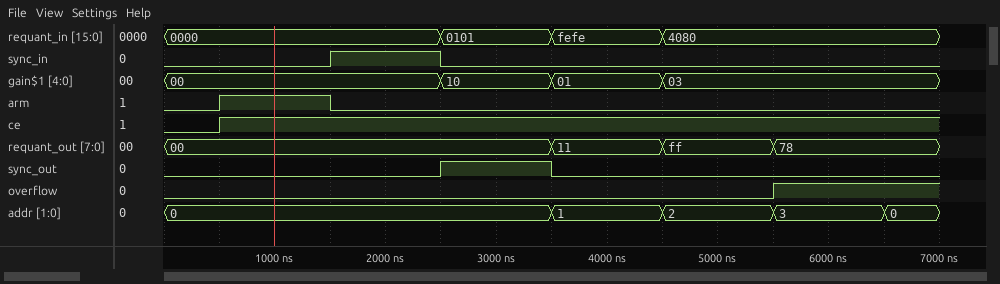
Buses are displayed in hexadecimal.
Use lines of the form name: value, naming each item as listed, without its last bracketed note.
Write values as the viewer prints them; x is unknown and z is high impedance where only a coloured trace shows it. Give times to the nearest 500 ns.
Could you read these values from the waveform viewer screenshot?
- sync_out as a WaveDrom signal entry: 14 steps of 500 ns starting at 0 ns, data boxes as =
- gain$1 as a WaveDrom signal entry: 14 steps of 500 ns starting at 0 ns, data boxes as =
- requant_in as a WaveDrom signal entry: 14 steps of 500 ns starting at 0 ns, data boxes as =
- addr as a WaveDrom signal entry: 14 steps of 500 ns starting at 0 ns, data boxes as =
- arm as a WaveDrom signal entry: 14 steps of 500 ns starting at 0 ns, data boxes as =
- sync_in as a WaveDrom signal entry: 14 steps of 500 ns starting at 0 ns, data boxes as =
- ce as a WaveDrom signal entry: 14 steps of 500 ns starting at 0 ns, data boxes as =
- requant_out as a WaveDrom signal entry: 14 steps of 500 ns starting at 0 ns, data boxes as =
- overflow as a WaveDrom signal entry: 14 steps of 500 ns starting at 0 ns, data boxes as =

sync_out as a WaveDrom signal entry: 14 steps of 500 ns starting at 0 ns, data boxes as =: {name: 'sync_out', wave: '0....1.0......'}
gain$1 as a WaveDrom signal entry: 14 steps of 500 ns starting at 0 ns, data boxes as =: {name: 'gain$1', wave: '=....=.=.=....', data: '00 10 01 03'}
requant_in as a WaveDrom signal entry: 14 steps of 500 ns starting at 0 ns, data boxes as =: {name: 'requant_in', wave: '=....=.=.=....', data: '0000 0101 fefe 4080'}
addr as a WaveDrom signal entry: 14 steps of 500 ns starting at 0 ns, data boxes as =: {name: 'addr', wave: '=......=.=.=.=', data: '0 1 2 3 0'}
arm as a WaveDrom signal entry: 14 steps of 500 ns starting at 0 ns, data boxes as =: {name: 'arm', wave: '01.0..........'}
sync_in as a WaveDrom signal entry: 14 steps of 500 ns starting at 0 ns, data boxes as =: {name: 'sync_in', wave: '0..1.0........'}
ce as a WaveDrom signal entry: 14 steps of 500 ns starting at 0 ns, data boxes as =: {name: 'ce', wave: '01............'}
requant_out as a WaveDrom signal entry: 14 steps of 500 ns starting at 0 ns, data boxes as =: {name: 'requant_out', wave: '=......=.=.=..', data: '00 11 ff 78'}
overflow as a WaveDrom signal entry: 14 steps of 500 ns starting at 0 ns, data boxes as =: {name: 'overflow', wave: '0..........1..'}
